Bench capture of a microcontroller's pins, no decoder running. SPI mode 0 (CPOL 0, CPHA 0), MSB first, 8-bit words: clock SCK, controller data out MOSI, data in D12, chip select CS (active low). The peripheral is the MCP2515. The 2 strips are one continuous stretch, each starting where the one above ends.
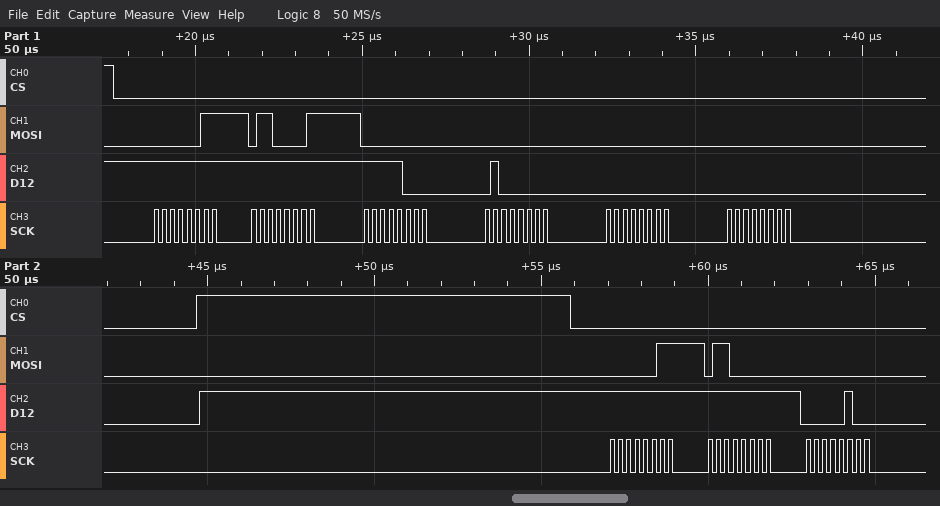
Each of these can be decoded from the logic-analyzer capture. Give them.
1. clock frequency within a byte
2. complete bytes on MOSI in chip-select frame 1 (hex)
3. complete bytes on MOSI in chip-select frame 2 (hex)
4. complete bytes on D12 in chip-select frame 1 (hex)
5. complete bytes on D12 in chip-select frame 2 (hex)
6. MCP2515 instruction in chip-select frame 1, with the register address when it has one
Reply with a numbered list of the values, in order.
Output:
1. 4 MHz
2. 03 61 00 00 00 00
3. 03 60 00
4. FF FF F8 40 00 00
5. FF FF 04
6. READ 0x61
